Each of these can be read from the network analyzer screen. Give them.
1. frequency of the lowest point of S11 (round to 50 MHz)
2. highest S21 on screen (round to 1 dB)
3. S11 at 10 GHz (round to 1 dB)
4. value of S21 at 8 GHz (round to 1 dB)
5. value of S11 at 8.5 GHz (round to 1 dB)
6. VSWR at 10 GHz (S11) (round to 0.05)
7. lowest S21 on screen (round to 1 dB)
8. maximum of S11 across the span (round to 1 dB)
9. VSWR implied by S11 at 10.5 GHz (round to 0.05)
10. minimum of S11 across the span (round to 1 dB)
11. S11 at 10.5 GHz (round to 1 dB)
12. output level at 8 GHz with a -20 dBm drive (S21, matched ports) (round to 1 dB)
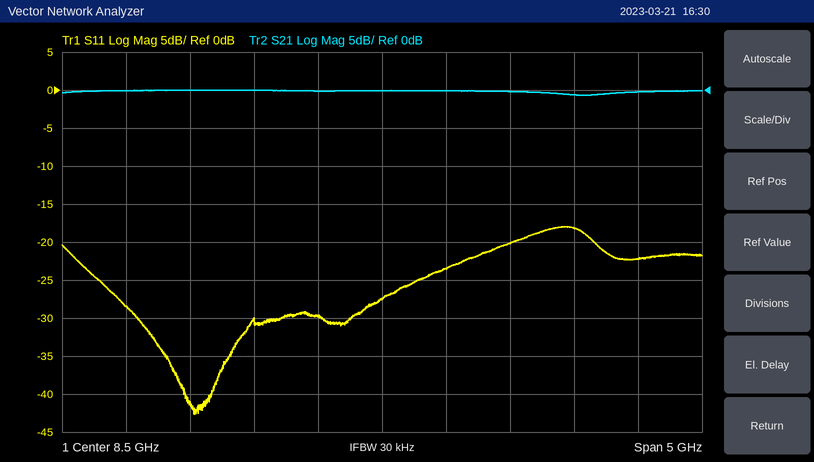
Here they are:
7.05 GHz
0 dB
-18 dB
0 dB
-27 dB
1.30
-1 dB
-18 dB
1.15
-43 dB
-22 dB
-20 dBm
